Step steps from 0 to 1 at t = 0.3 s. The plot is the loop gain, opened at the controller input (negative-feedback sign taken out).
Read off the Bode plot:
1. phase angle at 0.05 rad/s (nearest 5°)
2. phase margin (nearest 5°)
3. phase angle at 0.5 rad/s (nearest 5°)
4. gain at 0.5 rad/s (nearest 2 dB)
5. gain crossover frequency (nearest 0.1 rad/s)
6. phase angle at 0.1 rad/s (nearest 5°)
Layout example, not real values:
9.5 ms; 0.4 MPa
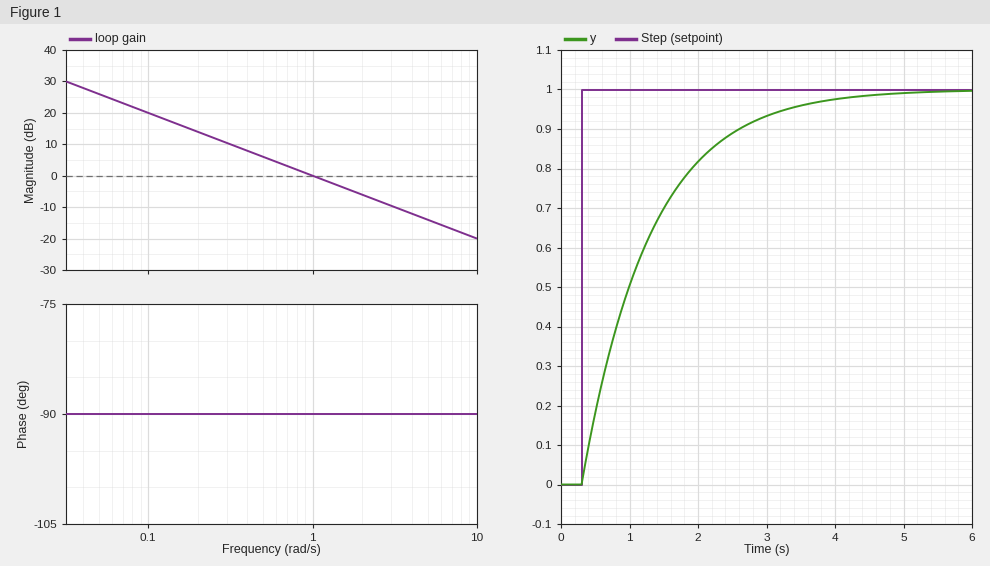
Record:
-90°; 90°; -90°; 6 dB; 1.0 rad/s; -90°
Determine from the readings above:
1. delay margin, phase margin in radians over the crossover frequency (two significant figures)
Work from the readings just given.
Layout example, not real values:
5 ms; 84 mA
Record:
1.6 s
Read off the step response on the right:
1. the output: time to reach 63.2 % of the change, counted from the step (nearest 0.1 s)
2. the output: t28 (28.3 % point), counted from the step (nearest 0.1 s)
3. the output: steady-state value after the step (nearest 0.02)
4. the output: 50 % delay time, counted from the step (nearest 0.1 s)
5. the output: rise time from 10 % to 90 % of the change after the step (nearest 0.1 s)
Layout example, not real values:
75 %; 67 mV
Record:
1.0 s; 0.3 s; 1.00; 0.7 s; 2.2 s
